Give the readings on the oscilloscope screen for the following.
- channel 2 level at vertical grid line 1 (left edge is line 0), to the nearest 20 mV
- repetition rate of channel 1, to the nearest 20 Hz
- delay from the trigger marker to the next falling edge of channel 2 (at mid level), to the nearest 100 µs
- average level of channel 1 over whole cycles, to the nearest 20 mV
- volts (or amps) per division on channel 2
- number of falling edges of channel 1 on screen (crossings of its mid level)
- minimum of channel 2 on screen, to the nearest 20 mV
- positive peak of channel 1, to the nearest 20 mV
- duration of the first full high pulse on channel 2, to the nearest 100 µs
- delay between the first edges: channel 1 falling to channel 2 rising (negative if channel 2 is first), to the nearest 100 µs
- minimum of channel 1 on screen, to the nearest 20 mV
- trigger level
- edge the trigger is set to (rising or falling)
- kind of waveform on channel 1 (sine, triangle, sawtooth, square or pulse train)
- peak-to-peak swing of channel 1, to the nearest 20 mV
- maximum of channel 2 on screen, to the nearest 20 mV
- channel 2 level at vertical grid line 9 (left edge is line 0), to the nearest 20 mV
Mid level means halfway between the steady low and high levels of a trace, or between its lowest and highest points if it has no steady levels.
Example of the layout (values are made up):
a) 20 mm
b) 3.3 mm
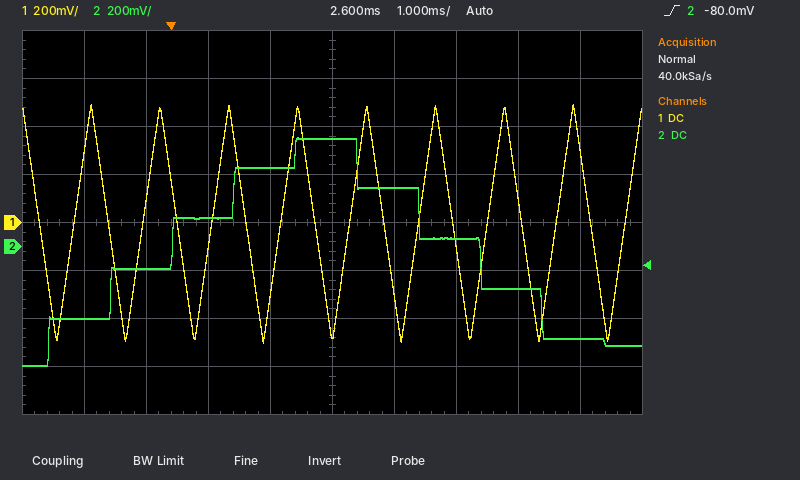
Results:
a) -300 mV
b) 900 Hz
c) 5.0 ms
d) 0 mV
e) 200 mV
f) 9
g) -500 mV
h) 500 mV
i) 5.0 ms
j) +2.1 ms
k) -500 mV
l) -80.0 mV
m) rising
n) triangle
o) 1.00 V
p) 460 mV
q) -380 mV
